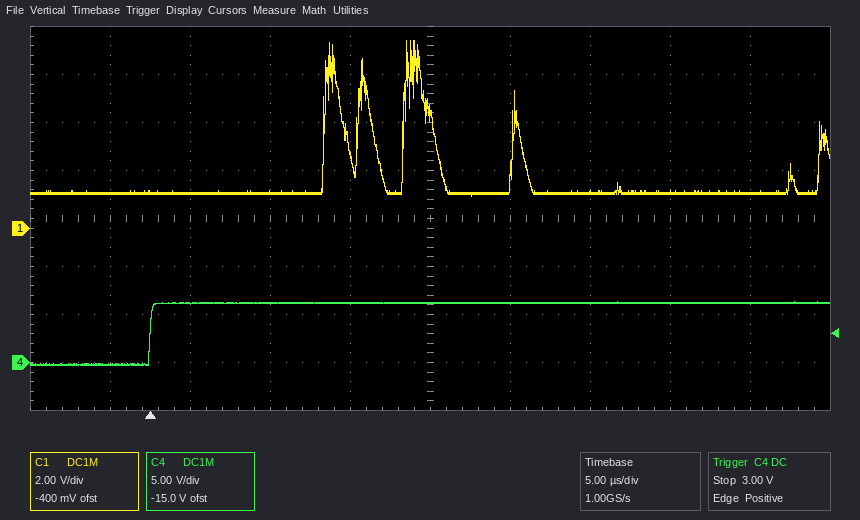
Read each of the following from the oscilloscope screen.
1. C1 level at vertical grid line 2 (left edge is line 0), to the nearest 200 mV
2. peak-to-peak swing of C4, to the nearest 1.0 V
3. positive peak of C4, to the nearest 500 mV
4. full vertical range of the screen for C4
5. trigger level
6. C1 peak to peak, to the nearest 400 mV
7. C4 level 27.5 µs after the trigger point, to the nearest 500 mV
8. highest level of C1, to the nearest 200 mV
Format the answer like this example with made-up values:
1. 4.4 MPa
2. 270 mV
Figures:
1. 1.4 V
2. 7.0 V
3. 6.5 V
4. 40 V
5. 3.00 V
6. 6.4 V
7. 6.0 V
8. 7.8 V
